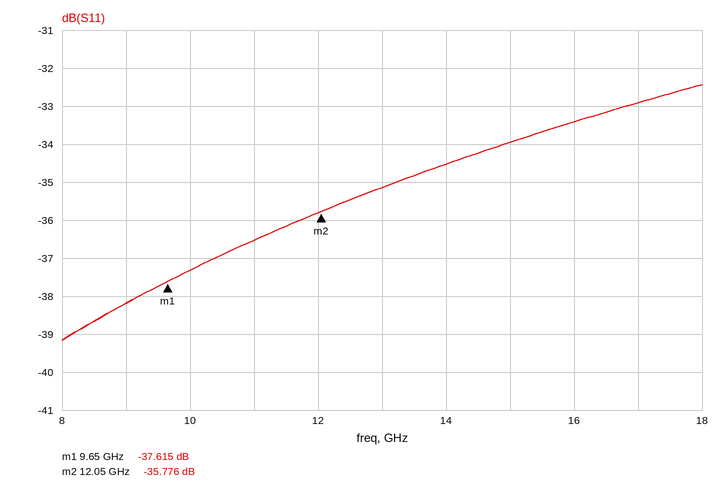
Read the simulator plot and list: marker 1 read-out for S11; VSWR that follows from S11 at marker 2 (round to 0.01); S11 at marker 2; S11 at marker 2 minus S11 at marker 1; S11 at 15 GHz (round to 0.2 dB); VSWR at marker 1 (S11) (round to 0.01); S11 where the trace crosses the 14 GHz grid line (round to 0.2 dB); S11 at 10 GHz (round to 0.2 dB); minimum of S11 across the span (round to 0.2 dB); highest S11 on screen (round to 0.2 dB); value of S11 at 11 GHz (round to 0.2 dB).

-37.615 dB
1.03
-35.776 dB
1.839 dB
-34.0 dB
1.03
-34.6 dB
-37.4 dB
-39.2 dB
-32.4 dB
-36.6 dB
